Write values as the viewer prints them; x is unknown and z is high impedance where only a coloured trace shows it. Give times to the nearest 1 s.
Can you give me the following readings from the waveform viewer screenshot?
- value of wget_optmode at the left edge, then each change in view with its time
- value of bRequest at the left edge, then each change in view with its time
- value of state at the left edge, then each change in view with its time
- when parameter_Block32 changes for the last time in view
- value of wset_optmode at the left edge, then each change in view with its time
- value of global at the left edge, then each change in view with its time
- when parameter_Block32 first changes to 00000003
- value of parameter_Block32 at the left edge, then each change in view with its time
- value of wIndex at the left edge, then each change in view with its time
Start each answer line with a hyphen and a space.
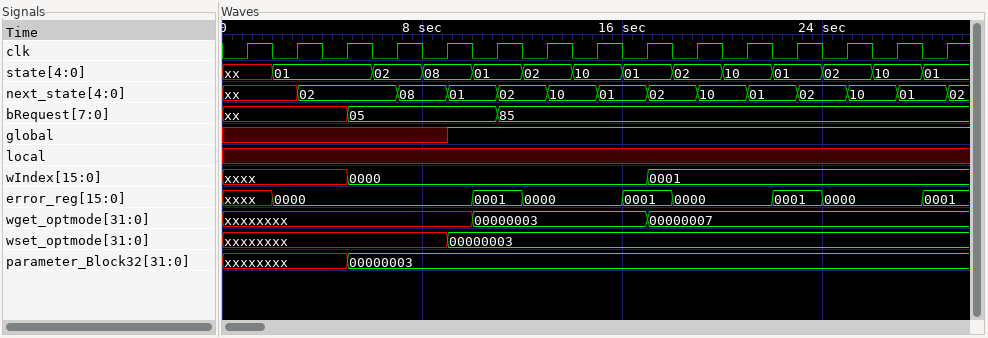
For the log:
- xxxxxxxx, 00000003 at 10 s, 00000007 at 17 s
- xx, 05 at 5 s, 85 at 11 s
- xx, 01 at 2 s, 02 at 6 s, 08 at 8 s, 01 at 10 s, 02 at 12 s, 10 at 14 s, 01 at 16 s, 02 at 18 s, 10 at 20 s, 01 at 22 s, 02 at 24 s, 10 at 26 s, 01 at 28 s
- 5 s
- xxxxxxxx, 00000003 at 9 s
- x, 1 at 9 s
- 5 s
- xxxxxxxx, 00000003 at 5 s
- xxxx, 0000 at 5 s, 0001 at 17 s
